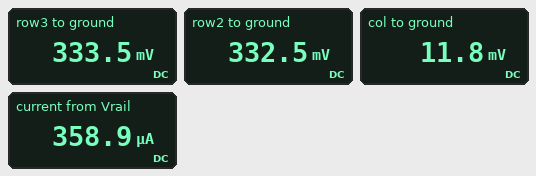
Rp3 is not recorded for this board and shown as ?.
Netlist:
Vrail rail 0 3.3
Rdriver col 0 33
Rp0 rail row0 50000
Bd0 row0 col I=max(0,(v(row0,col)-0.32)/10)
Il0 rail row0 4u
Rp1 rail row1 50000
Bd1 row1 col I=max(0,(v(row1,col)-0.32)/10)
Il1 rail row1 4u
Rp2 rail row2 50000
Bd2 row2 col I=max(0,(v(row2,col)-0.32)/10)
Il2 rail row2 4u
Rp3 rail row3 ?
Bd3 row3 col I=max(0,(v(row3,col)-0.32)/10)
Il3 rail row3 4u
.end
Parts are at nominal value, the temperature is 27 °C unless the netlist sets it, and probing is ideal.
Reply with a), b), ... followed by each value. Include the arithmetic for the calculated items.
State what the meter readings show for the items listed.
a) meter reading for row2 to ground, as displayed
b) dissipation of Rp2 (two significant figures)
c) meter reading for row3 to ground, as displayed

a) 332.5 mV
b) (3.3 V - 332.5 mV)^2 / 50 kΩ = 180 µW
c) 333.5 mV
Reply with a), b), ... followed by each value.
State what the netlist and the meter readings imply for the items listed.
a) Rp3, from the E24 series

a) 18 kΩ
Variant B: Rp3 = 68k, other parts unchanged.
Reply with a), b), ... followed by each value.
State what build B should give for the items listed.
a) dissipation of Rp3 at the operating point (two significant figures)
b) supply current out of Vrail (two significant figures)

a) 130 µW
b) 240 µA
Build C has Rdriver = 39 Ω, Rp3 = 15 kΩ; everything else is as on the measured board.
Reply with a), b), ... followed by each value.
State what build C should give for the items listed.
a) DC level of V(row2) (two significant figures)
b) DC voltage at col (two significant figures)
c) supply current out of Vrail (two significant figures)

a) 340 mV
b) 15 mV
c) 390 µA
